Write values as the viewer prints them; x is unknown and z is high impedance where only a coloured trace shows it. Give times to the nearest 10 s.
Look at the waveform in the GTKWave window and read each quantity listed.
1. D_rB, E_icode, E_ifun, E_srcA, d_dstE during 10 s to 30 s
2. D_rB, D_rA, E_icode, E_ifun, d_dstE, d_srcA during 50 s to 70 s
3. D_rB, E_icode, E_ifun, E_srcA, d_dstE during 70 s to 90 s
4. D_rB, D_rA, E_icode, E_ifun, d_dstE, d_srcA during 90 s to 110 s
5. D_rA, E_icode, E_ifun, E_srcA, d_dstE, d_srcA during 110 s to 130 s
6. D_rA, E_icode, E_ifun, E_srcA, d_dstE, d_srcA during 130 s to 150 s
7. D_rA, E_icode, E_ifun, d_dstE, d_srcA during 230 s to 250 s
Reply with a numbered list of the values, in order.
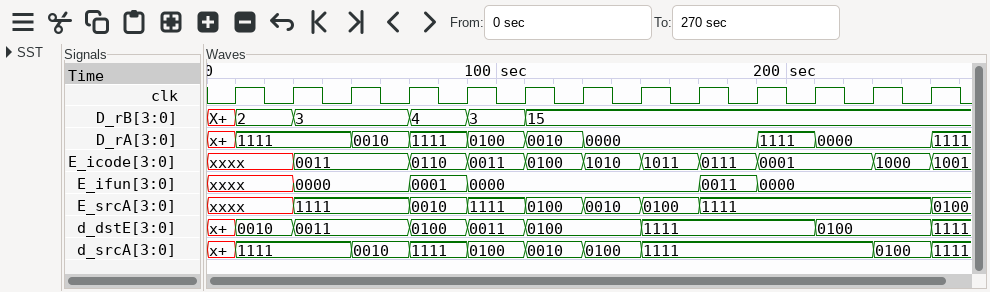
1. D_rB=2, E_icode=xxxx, E_ifun=xxxx, E_srcA=xxxx, d_dstE=0010
2. D_rB=3, D_rA=0010, E_icode=0011, E_ifun=0000, d_dstE=0011, d_srcA=0010
3. D_rB=4, E_icode=0110, E_ifun=0001, E_srcA=0010, d_dstE=0100
4. D_rB=3, D_rA=0100, E_icode=0011, E_ifun=0000, d_dstE=0011, d_srcA=0100
5. D_rA=0010, E_icode=0100, E_ifun=0000, E_srcA=0100, d_dstE=0100, d_srcA=0010
6. D_rA=0000, E_icode=1010, E_ifun=0000, E_srcA=0010, d_dstE=0100, d_srcA=0100
7. D_rA=0000, E_icode=1000, E_ifun=0000, d_dstE=0100, d_srcA=0100
